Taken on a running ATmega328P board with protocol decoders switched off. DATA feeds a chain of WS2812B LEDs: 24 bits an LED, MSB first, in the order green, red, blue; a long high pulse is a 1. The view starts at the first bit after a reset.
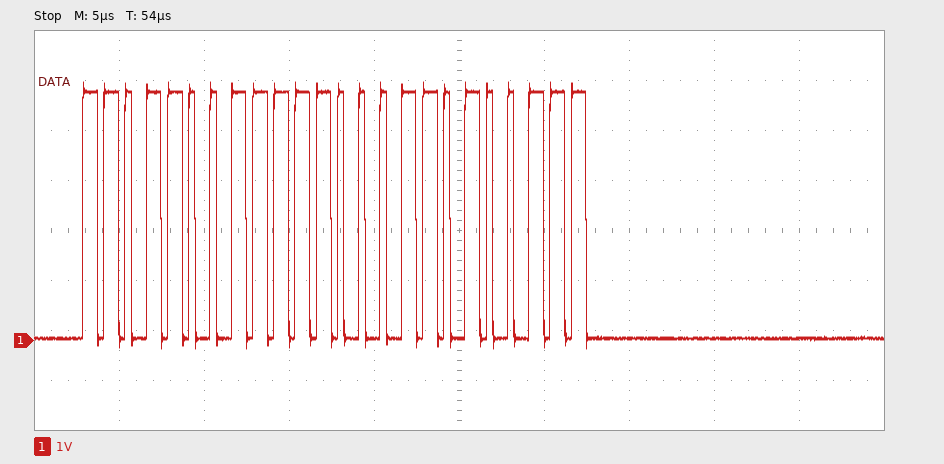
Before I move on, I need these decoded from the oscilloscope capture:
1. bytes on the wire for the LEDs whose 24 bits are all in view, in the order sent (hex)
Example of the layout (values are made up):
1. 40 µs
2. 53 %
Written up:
1. D9 F1 A7
